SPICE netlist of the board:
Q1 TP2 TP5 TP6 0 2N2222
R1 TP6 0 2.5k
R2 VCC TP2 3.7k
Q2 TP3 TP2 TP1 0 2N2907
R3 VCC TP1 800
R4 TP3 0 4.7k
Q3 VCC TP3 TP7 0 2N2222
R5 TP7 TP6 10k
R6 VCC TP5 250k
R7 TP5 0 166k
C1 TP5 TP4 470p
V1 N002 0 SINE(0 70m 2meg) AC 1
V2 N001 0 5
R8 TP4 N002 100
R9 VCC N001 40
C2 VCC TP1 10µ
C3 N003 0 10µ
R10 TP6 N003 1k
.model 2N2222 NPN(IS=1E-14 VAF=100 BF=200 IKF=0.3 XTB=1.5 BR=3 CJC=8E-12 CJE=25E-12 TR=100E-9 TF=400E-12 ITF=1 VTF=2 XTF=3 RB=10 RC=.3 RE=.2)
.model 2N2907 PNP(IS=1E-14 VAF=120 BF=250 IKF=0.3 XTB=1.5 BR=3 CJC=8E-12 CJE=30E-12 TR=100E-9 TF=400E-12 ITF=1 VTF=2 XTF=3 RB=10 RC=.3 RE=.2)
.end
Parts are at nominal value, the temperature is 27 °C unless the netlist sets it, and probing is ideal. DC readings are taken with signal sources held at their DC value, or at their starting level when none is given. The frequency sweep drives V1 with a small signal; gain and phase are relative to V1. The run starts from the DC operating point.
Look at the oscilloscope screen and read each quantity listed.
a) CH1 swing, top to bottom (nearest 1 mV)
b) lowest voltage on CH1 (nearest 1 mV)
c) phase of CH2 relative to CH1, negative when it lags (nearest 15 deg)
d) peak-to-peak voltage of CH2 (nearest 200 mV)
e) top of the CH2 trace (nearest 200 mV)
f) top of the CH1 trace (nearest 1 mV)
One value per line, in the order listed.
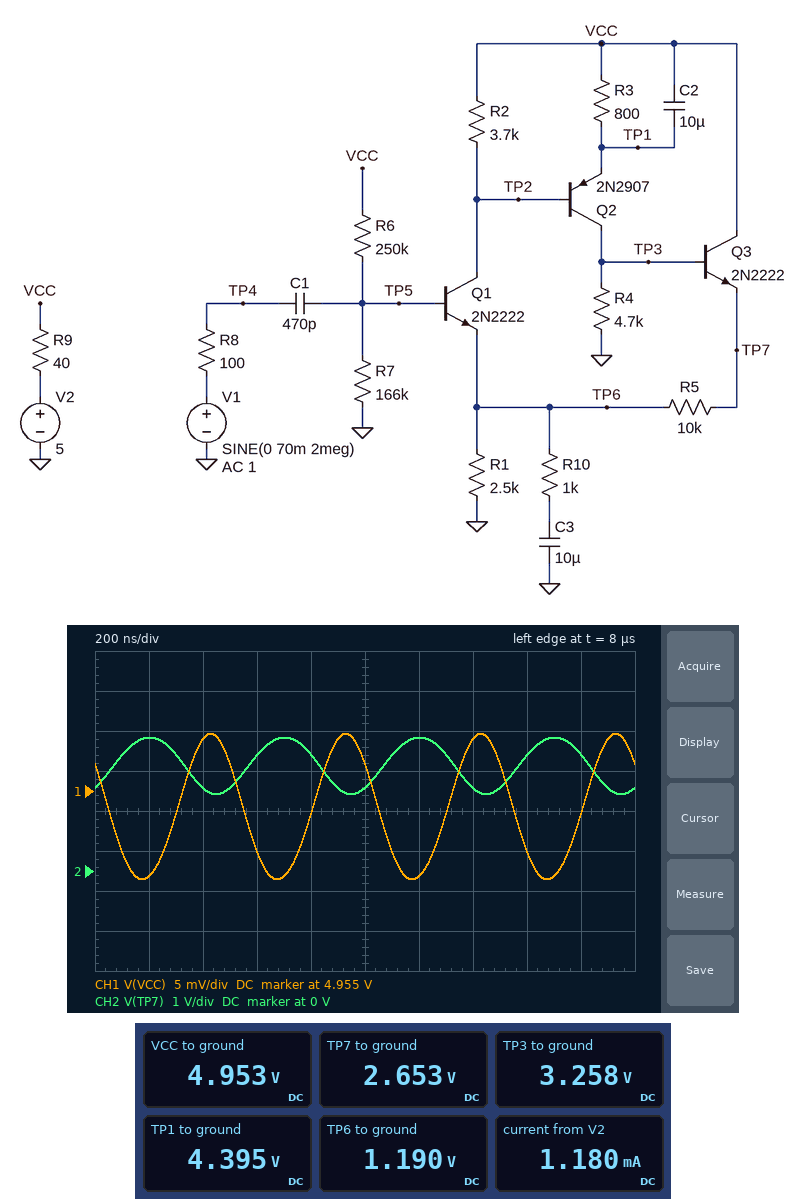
18 mV
4.944 V
165 deg
1.4 V
3.4 V
4.962 V
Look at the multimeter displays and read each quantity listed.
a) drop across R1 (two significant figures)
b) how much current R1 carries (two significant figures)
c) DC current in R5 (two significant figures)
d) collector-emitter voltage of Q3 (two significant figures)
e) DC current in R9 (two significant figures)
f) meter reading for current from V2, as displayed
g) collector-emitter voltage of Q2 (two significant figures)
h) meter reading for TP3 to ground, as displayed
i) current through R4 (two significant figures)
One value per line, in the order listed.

1.2 V
480 µA
150 µA
2.3 V
1.2 mA
1.180 mA
-1.1 V
3.258 V
690 µA
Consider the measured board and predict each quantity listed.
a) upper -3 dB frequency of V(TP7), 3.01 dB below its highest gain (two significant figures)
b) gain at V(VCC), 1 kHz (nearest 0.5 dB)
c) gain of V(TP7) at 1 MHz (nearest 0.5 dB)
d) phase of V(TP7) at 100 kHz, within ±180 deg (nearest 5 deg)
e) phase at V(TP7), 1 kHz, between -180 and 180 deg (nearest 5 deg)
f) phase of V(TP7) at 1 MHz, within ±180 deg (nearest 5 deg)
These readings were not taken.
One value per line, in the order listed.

2.1 MHz
-26.5 dB
22.0 dB
0 deg
75 deg
-30 deg
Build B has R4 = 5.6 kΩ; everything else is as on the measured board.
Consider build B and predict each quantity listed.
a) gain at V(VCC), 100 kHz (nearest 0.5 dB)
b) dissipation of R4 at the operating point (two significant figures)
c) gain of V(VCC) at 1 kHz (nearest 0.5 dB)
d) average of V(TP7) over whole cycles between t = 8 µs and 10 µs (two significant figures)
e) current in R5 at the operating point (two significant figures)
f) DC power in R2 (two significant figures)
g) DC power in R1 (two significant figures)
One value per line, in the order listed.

-16.0 dB
2.2 mW
-27.5 dB
2.9 V
170 µA
350 µW
580 µW
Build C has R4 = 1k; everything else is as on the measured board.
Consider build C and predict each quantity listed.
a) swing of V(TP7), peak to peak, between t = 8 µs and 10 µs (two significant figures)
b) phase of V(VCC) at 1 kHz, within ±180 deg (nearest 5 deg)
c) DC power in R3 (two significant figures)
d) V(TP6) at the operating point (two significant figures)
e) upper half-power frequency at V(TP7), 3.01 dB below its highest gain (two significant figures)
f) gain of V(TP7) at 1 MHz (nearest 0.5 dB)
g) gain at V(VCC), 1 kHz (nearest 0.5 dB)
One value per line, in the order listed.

1.2 V
-85 deg
1.2 mW
1.1 V
3.0 MHz
20.0 dB
-8.0 dB
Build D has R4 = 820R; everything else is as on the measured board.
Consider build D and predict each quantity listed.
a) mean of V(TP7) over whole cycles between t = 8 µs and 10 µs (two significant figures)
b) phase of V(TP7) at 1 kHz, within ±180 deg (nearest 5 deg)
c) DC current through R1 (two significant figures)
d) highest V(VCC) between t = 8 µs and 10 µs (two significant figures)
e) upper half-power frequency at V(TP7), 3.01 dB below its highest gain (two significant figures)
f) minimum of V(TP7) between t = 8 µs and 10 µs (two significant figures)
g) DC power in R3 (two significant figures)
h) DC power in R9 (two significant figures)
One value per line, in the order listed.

1.1 V
80 deg
450 µA
5.0 V
3.0 MHz
550 mV
1.2 mW
110 µW
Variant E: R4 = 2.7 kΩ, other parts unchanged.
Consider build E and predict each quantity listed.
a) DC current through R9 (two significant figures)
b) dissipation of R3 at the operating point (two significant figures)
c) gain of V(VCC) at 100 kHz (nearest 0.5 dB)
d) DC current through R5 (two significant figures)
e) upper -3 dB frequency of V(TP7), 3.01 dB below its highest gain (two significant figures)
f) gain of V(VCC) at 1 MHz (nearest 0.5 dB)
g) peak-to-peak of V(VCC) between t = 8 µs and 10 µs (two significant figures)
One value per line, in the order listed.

1.4 mA
700 µW
-11.5 dB
77 µA
2.2 MHz
-12.0 dB
28 mV
